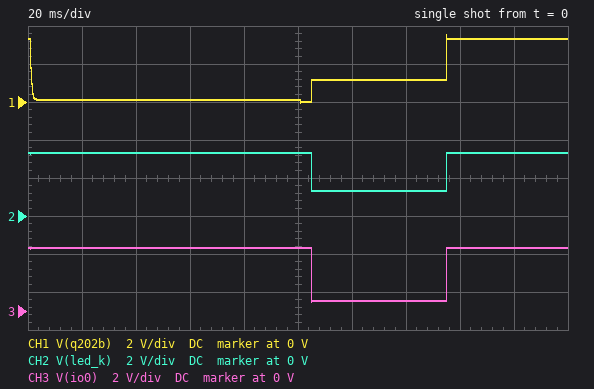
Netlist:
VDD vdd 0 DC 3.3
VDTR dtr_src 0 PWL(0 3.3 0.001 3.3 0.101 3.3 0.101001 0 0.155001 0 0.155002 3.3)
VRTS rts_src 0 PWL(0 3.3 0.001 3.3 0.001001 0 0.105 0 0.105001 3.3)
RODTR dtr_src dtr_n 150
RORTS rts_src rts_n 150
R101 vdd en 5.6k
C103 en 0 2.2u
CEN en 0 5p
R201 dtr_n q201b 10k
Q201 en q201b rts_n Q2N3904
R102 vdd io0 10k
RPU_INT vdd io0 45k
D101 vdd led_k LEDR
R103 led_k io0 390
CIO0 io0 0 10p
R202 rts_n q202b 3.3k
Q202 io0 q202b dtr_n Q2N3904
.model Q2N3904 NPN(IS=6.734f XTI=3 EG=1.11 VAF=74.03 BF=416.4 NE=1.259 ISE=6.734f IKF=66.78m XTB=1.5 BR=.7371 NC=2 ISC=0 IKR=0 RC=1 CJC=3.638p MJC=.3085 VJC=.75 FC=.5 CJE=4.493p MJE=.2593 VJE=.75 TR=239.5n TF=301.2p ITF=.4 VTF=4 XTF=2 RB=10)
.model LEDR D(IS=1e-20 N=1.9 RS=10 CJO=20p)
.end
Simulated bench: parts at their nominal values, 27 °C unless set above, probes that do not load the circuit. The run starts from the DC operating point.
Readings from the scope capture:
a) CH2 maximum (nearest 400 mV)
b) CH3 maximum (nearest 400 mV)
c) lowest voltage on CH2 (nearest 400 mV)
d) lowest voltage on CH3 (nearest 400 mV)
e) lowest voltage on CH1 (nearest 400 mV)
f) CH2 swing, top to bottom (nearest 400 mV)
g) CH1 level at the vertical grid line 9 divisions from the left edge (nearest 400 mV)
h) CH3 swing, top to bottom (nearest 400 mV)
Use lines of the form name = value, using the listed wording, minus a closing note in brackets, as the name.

CH2 maximum = 3.2 V
CH3 maximum = 3.2 V
lowest voltage on CH2 = 1.2 V
lowest voltage on CH3 = 400 mV
lowest voltage on CH1 = 0 V
CH2 swing, top to bottom = 2.0 V
CH1 level at the vertical grid line 9 divisions from the left edge = 3.2 V
CH3 swing, top to bottom = 2.8 V
